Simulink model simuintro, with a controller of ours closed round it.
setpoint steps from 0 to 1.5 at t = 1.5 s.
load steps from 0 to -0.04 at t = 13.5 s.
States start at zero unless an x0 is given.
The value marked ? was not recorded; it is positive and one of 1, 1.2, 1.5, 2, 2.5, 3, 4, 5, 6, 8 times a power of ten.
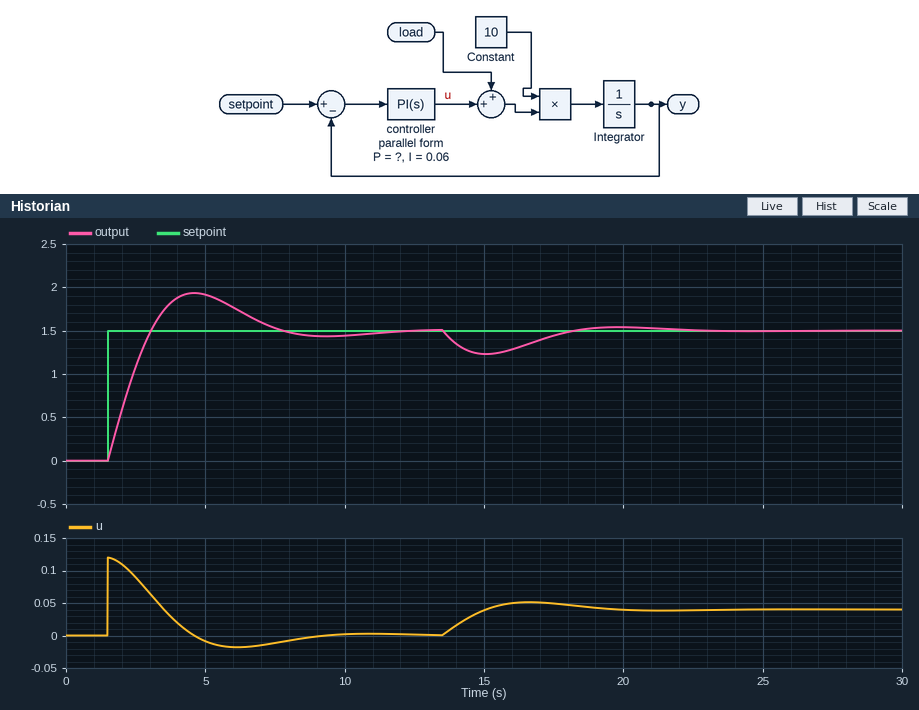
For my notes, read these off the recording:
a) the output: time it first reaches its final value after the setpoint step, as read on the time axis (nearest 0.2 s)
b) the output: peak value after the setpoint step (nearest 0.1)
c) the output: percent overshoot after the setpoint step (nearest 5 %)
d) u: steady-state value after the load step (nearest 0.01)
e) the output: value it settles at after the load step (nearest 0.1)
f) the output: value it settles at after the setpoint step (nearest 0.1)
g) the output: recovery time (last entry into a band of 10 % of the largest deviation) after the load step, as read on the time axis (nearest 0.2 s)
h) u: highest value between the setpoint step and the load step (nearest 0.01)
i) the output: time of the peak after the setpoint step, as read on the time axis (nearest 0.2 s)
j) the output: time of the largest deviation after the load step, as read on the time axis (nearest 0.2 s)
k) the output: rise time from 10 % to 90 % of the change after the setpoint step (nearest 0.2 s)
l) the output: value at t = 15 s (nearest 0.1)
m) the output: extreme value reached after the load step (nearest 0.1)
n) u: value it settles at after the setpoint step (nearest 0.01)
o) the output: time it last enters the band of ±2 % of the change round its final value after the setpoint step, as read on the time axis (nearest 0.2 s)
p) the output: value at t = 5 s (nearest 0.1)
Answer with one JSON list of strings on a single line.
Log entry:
["3.0 s", "1.9", "30 %", "0.04", "1.5", "1.5", "21.0 s", "0.12", "4.6 s", "15.0 s", "1.2 s", "1.2", "1.2", "0.00", "11.2 s", "1.9"]
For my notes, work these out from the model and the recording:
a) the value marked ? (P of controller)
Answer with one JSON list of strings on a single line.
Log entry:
["0.08"]
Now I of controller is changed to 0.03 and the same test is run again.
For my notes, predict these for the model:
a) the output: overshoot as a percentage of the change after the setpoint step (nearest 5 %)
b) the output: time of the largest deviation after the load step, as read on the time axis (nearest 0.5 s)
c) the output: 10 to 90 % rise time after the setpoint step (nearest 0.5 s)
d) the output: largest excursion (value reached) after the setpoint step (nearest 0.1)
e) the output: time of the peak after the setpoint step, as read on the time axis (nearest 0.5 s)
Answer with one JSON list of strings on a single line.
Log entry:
["20 %", "15.5 s", "1.5 s", "1.8", "5.5 s"]
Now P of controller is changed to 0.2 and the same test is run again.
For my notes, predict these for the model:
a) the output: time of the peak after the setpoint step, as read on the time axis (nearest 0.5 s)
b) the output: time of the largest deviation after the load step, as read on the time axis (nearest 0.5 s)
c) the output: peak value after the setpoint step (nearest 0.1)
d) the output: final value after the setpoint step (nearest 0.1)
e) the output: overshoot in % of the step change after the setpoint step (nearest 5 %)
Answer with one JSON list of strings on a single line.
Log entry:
["4.0 s", "14.5 s", "1.6", "1.5", "10 %"]
